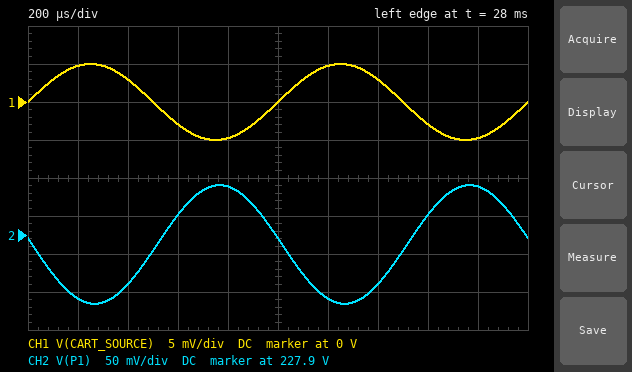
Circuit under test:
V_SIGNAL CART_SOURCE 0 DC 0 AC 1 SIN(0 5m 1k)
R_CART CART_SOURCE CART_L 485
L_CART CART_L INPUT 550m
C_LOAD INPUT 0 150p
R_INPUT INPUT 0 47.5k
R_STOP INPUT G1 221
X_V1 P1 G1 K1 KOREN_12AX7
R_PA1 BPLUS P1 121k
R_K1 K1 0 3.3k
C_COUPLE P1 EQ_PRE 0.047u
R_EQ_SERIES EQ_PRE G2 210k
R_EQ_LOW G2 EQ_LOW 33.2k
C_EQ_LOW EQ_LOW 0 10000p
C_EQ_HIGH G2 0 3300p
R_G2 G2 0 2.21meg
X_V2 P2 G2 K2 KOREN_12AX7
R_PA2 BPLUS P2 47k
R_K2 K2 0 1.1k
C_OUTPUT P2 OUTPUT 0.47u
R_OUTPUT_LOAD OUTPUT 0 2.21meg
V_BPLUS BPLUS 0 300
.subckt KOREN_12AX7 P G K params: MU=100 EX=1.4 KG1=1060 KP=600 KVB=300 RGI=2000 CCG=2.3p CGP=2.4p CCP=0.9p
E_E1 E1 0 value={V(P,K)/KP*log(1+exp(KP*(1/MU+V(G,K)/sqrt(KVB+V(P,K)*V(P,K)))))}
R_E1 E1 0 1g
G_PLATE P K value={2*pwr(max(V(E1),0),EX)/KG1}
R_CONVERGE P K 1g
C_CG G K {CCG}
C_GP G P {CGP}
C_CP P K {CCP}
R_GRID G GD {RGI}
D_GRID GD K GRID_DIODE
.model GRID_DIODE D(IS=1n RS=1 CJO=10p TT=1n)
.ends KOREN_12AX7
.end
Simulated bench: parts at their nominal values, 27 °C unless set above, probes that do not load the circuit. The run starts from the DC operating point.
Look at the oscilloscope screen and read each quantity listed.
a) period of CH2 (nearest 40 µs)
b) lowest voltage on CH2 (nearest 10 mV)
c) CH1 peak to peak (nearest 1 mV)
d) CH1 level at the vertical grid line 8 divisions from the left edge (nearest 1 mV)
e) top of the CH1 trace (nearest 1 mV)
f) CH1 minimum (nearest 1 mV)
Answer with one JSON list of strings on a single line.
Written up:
["1.00 ms", "227.81 V", "10 mV", "-3 mV", "5 mV", "-5 mV"]
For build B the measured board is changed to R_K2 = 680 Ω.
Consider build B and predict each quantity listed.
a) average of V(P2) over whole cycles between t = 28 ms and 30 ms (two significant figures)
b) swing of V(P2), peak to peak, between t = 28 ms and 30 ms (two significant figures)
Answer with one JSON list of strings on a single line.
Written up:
["220 V", "490 mV"]
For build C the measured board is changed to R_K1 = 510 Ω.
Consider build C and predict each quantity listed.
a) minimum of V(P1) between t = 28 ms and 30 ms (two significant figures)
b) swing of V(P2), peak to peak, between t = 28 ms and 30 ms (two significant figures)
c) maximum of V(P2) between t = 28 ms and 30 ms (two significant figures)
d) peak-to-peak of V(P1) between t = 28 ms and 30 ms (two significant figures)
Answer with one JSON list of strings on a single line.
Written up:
["140 V", "1.1 V", "230 V", "440 mV"]
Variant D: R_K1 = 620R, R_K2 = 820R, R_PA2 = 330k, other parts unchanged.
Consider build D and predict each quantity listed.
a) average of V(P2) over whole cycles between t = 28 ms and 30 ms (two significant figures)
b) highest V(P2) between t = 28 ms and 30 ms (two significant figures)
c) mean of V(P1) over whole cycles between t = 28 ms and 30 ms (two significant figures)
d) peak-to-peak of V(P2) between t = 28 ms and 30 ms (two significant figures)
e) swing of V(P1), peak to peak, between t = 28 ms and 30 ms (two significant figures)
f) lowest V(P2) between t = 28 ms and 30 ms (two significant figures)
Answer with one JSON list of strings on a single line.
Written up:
["95 V", "96 V", "150 V", "2.9 V", "410 mV", "93 V"]
